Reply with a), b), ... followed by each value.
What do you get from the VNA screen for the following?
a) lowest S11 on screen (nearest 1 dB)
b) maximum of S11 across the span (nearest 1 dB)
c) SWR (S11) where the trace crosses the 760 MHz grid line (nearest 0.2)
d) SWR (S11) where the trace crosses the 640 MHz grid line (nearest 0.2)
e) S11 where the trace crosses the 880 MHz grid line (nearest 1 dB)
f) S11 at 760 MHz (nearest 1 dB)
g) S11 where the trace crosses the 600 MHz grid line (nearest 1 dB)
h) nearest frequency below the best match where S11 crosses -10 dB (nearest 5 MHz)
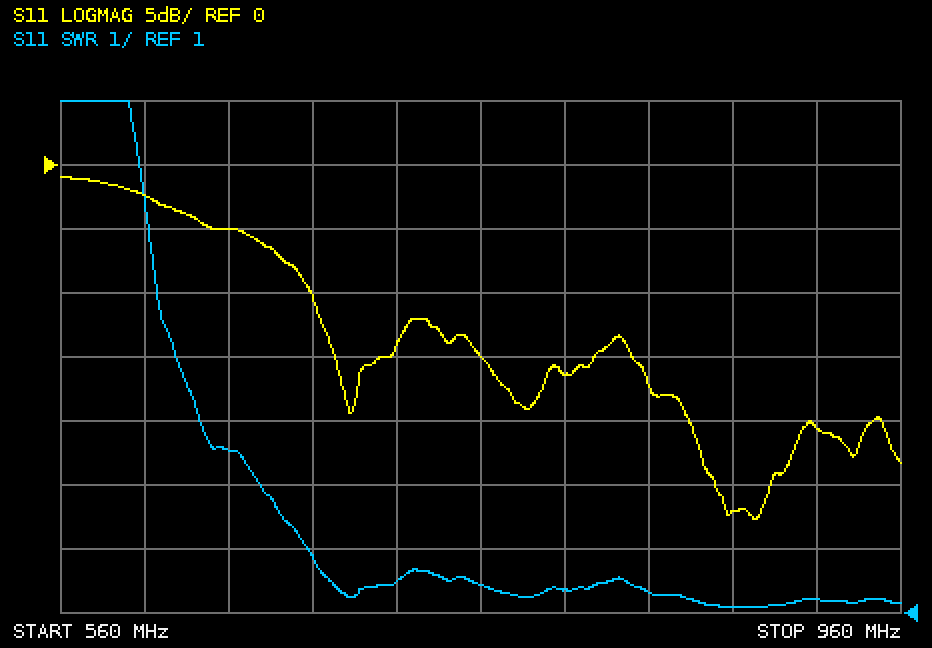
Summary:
a) -28 dB
b) -1 dB
c) 1.4
d) 3.6
e) -27 dB
f) -15 dB
g) -2 dB
h) 680 MHz
